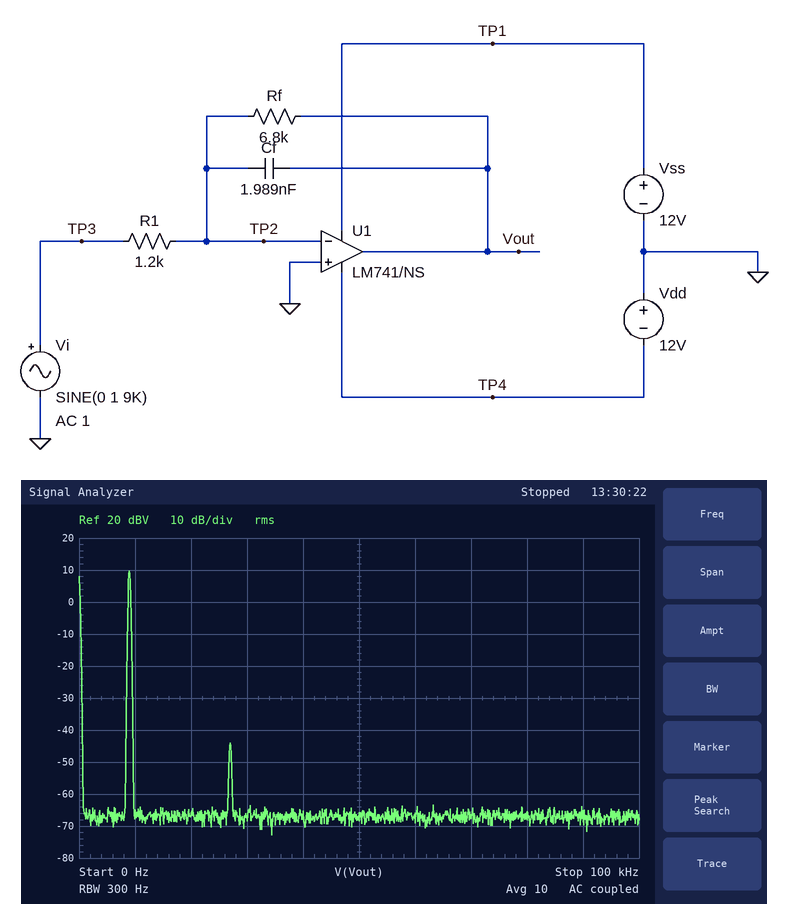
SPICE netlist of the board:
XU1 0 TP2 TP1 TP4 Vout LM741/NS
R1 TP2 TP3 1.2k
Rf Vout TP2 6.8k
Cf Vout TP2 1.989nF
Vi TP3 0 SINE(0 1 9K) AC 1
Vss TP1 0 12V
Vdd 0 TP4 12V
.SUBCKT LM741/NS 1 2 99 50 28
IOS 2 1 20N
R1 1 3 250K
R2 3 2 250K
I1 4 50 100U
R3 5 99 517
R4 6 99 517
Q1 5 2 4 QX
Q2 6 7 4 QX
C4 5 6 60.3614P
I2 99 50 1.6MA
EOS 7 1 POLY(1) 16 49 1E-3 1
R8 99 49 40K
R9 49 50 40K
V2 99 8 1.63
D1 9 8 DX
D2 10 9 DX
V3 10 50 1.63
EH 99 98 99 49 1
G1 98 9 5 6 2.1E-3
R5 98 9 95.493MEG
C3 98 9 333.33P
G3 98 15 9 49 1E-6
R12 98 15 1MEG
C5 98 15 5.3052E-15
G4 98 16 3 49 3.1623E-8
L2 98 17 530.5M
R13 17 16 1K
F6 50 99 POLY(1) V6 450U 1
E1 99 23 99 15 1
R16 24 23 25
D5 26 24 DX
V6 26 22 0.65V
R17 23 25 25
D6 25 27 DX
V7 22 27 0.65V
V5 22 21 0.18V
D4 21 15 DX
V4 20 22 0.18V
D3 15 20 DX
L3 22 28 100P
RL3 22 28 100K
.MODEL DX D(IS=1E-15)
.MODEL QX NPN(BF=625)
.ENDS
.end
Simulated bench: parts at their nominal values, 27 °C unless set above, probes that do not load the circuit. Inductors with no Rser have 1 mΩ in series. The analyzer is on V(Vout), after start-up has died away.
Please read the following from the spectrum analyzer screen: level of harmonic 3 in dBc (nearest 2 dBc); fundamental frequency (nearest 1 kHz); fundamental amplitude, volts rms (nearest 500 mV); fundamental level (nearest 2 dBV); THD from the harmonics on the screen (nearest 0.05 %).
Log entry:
-54 dBc
9 kHz
3.0 V
10 dBV
0.20 %
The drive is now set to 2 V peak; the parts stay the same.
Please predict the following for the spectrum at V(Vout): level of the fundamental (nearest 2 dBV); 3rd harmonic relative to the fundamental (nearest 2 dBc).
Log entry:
14 dBV
-24 dBc
